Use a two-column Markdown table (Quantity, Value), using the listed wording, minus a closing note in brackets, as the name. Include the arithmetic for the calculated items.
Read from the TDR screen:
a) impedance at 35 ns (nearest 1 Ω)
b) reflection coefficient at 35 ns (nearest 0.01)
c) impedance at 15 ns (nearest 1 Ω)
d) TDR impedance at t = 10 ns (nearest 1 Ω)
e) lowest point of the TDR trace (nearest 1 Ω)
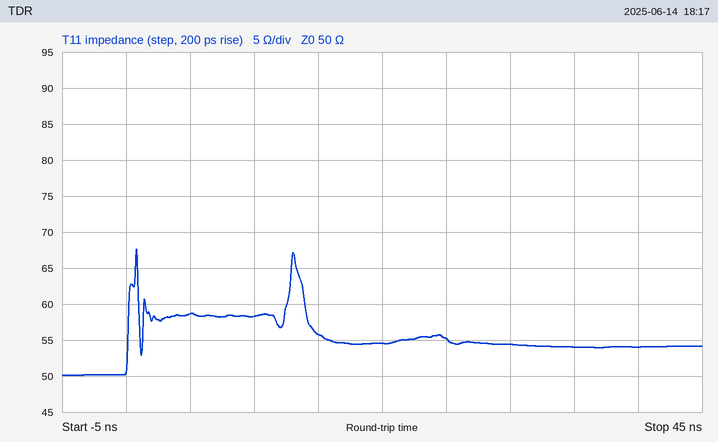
| Quantity | Value |
|---|---|
| impedance at 35 ns | 54 Ω |
| reflection coefficient at 35 ns | (54 − 50)/(54 + 50) ≈ +0.04 |
| impedance at 15 ns | 56 Ω |
| TDR impedance at t = 10 ns | 58 Ω |
| lowest point of the TDR trace | 50 Ω |
